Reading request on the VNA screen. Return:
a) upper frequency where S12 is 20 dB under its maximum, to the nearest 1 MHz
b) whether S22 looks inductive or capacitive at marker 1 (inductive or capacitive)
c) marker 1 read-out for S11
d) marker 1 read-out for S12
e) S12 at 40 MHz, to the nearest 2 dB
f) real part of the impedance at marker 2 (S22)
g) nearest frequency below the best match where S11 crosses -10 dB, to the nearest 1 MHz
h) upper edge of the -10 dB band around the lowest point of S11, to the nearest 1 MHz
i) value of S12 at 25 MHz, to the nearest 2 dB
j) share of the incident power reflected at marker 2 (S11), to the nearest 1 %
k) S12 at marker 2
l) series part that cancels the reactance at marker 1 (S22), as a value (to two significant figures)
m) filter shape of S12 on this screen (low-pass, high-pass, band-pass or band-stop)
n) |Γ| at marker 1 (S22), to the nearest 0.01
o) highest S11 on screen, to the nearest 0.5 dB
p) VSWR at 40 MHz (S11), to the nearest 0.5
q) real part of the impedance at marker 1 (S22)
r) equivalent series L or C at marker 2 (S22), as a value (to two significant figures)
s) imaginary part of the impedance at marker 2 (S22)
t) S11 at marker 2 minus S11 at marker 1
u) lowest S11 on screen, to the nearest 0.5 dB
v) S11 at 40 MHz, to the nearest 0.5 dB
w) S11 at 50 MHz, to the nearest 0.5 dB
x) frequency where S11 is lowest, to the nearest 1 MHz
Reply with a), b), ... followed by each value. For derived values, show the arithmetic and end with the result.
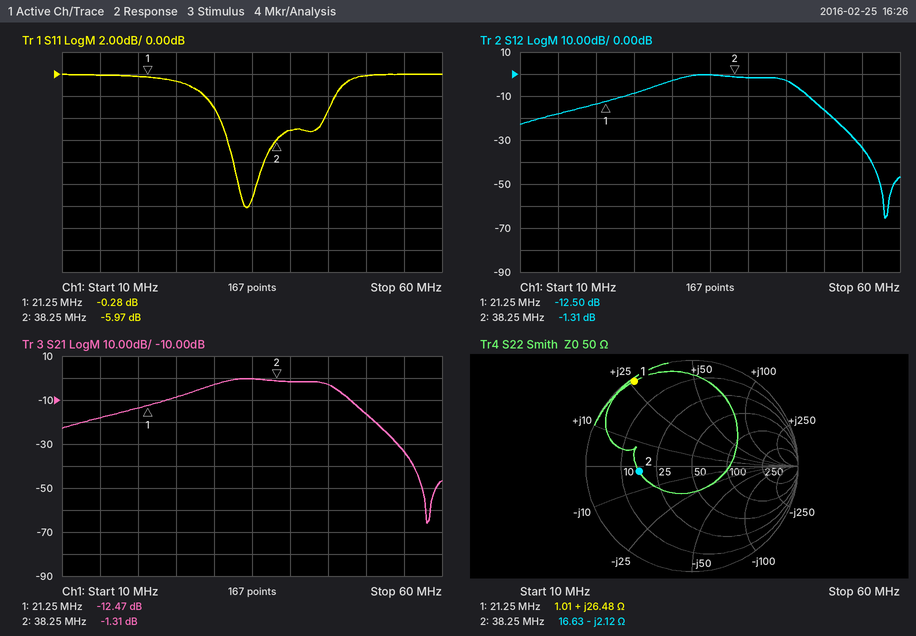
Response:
a) 51 MHz
b) inductive
c) -0.28 dB
d) -12.50 dB
e) -2 dB
f) 16.63 Ω
g) 33 MHz
h) 36 MHz
i) -8 dB
j) 10^(-5.97/10) ≈ 25 %
k) -1.31 dB
l) C = 1/(2π × 21.25 MHz × 26.48 Ω) ≈ 283 pF, so 280 pF to two significant figures
m) band-pass
n) 0.97
o) 0.0 dB
p) |Γ| = 10^(-5/20) = 0.5623; VSWR = (1 + 0.5623)/(1 − 0.5623) ≈ 3.57, so 3.5 to the nearest 0.5
q) 1.01 Ω
r) C = 1/(2π × 38.25 MHz × 2.12 Ω) ≈ 2.0 nF
s) -2.12 Ω
t) -5.97 − (-0.28) = -5.69 dB
u) -12.0 dB
v) -5.0 dB
w) 0.0 dB
x) 34 MHz
